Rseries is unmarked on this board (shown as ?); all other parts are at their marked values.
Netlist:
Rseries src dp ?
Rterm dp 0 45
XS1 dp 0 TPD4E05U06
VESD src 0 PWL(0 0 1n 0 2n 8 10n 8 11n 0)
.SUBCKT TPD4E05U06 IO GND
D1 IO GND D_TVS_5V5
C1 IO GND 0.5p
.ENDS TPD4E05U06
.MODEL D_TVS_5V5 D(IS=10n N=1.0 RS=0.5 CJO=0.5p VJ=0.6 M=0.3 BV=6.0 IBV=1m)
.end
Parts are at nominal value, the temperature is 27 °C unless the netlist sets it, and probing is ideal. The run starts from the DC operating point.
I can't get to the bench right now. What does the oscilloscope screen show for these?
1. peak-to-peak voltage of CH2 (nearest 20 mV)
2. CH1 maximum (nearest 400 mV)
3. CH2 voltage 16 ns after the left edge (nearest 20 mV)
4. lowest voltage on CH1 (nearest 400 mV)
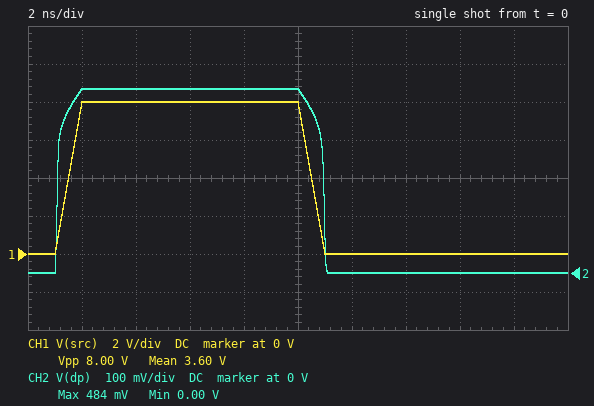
480 mV
8.0 V
0 V
0 V
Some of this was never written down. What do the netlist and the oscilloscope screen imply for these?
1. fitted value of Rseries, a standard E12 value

56 Ω
